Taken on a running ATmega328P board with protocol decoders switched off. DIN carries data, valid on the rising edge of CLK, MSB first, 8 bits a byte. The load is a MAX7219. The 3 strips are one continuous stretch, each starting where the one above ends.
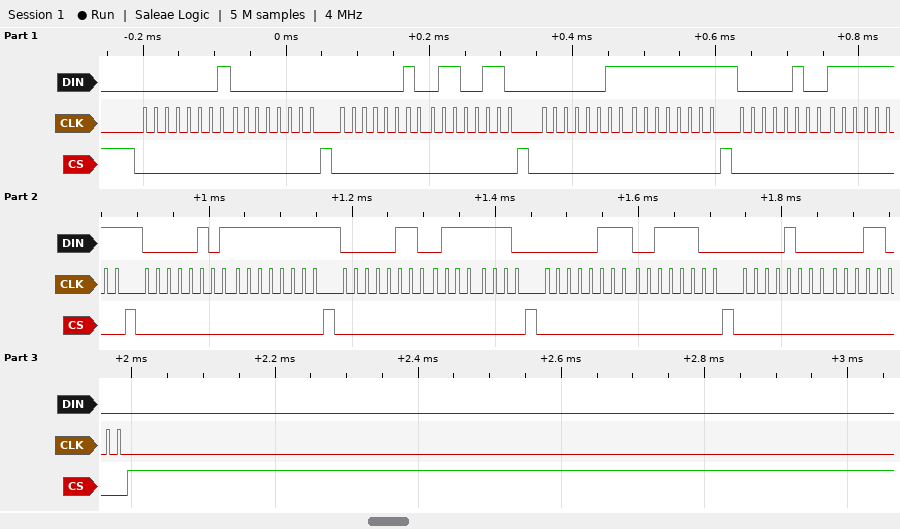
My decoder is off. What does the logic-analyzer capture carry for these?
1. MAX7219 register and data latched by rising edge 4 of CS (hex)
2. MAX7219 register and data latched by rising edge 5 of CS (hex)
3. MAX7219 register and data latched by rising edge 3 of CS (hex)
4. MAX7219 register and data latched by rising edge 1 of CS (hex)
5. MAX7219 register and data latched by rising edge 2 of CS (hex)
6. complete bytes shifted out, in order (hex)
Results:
register 0x4, data 0xFF
register 0x5, data 0xFF
register 0x3, data 0xFF
register 0x1, data 0x00
register 0x2, data 0x66
01 00 02 66 03 FF 04 FF 05 FF 06 7E 07 3C 08 18
